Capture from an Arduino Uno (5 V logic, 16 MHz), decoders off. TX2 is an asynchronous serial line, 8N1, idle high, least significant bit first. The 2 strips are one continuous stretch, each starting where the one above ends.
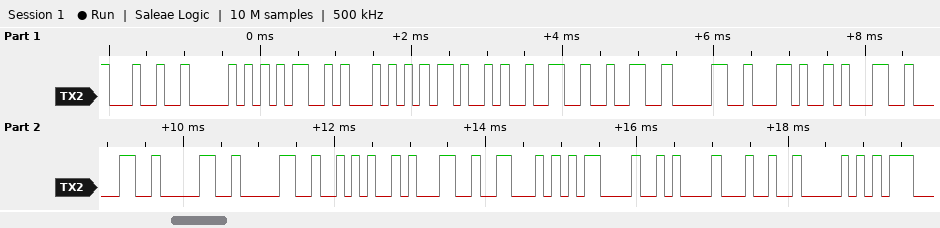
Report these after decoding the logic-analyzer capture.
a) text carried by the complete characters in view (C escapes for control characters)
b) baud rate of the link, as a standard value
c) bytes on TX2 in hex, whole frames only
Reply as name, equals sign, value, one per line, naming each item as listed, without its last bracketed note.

text carried by the complete characters in view = "$PMTK220,1000*1F\r\n$P"
baud rate of the link, as a standard value = 9600 baud
bytes on TX2 in hex, whole frames only = 24 50 4D 54 4B 32 32 30 2C 31 30 30 30 2A 31 46 0D 0A 24 50
